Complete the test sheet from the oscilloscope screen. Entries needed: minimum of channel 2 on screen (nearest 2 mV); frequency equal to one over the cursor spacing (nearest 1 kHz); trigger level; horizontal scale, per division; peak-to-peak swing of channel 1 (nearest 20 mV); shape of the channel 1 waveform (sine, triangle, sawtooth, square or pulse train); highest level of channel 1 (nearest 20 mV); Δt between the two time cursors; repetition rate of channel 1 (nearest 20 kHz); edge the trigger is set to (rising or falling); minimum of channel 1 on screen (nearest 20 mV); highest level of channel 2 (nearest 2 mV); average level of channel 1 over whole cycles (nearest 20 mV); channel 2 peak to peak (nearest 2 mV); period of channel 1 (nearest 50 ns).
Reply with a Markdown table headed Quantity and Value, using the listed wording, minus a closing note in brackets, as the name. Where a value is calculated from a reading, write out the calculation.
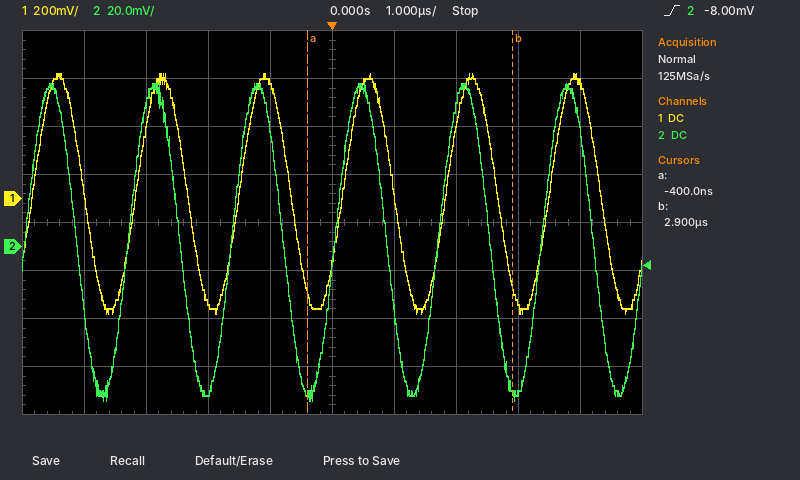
| Quantity | Value |
|---|---|
| minimum of channel 2 on screen | -64 mV |
| frequency equal to one over the cursor spacing | 1 / 3.3 µs ≈ 303 kHz |
| trigger level | -8.00 mV |
| horizontal scale, per division | 1 µs |
| peak-to-peak swing of channel 1 | 520 mV − (-480 mV) = 1.00 V |
| shape of the channel 1 waveform | sine |
| highest level of channel 1 | 520 mV |
| Δt between the two time cursors | 2.9 µs − (-400 ns) = 3.3 µs |
| repetition rate of channel 1 | 1 / 1.65 µs ≈ 606 kHz, so 600 kHz to the nearest 20 kHz |
| edge the trigger is set to | rising |
| minimum of channel 1 on screen | -480 mV |
| highest level of channel 2 | 68 mV |
| average level of channel 1 over whole cycles | (520 mV + (-480 mV)) / 2 ≈ 20 mV |
| channel 2 peak to peak | 68 mV − (-64 mV) = 132 mV |
| period of channel 1 | 1.65 µs |
